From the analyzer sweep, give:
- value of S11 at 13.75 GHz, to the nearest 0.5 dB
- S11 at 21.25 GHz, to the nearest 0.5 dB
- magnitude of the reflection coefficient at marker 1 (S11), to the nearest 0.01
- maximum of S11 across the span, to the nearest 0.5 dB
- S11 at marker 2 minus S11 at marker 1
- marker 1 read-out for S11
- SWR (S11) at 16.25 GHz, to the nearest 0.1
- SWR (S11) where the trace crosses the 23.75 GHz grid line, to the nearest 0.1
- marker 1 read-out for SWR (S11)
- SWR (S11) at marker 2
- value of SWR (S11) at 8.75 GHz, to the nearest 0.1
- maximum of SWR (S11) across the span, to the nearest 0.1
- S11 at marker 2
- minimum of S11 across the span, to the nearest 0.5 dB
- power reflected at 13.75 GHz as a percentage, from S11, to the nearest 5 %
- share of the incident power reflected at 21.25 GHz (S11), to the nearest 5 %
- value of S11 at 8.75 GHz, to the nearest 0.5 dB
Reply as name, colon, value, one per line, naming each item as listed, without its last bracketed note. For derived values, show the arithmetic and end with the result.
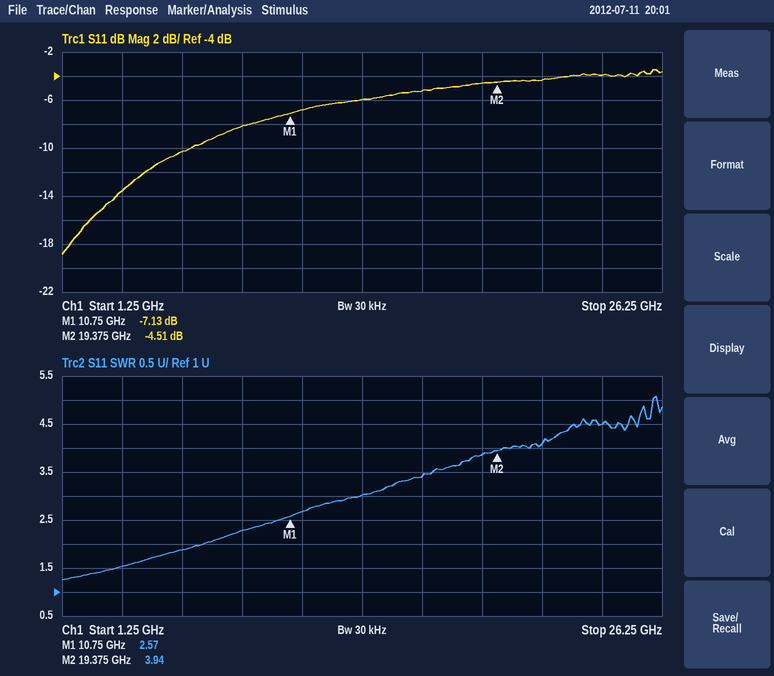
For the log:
value of S11 at 13.75 GHz, to the nearest 0.5 dB: -6.0 dB
S11 at 21.25 GHz, to the nearest 0.5 dB: -4.5 dB
magnitude of the reflection coefficient at marker 1 (S11), to the nearest 0.01: 10^(-7.13/20) ≈ 0.44
maximum of S11 across the span, to the nearest 0.5 dB: -3.5 dB
S11 at marker 2 minus S11 at marker 1: -4.51 − (-7.13) = 2.62 dB
marker 1 read-out for S11: -7.13 dB
SWR (S11) at 16.25 GHz, to the nearest 0.1: 3.4
SWR (S11) where the trace crosses the 23.75 GHz grid line, to the nearest 0.1: 4.5
marker 1 read-out for SWR: 2.57
SWR (S11) at marker 2: 3.94
value of SWR (S11) at 8.75 GHz, to the nearest 0.1: 2.3
maximum of SWR (S11) across the span, to the nearest 0.1: 5.1
S11 at marker 2: -4.51 dB
minimum of S11 across the span, to the nearest 0.5 dB: -19.0 dB
power reflected at 13.75 GHz as a percentage, from S11, to the nearest 5 %: 10^(-6/10) ≈ 25 %
share of the incident power reflected at 21.25 GHz (S11), to the nearest 5 %: 10^(-4.5/10) ≈ 35 %
value of S11 at 8.75 GHz, to the nearest 0.5 dB: -8.0 dB
